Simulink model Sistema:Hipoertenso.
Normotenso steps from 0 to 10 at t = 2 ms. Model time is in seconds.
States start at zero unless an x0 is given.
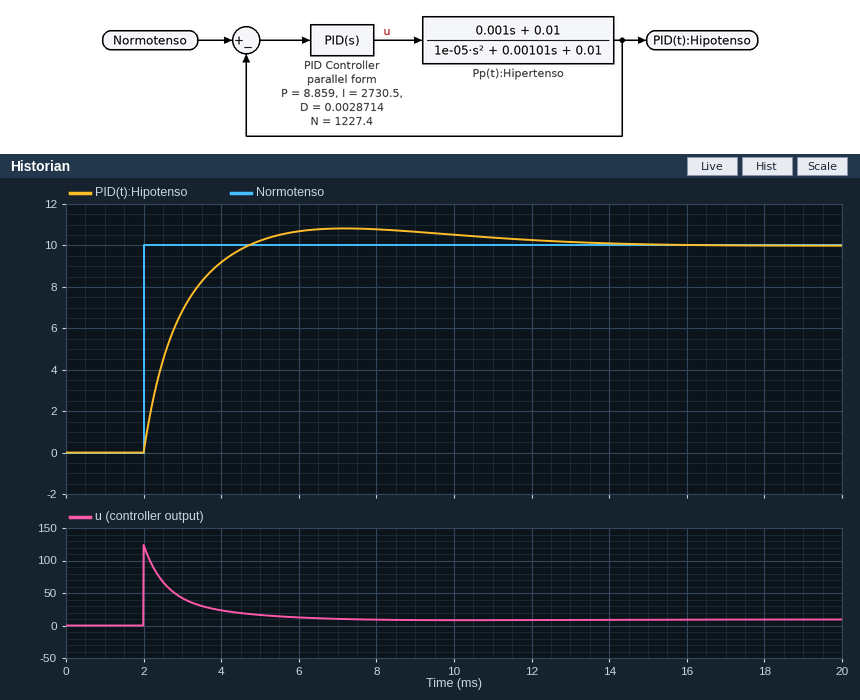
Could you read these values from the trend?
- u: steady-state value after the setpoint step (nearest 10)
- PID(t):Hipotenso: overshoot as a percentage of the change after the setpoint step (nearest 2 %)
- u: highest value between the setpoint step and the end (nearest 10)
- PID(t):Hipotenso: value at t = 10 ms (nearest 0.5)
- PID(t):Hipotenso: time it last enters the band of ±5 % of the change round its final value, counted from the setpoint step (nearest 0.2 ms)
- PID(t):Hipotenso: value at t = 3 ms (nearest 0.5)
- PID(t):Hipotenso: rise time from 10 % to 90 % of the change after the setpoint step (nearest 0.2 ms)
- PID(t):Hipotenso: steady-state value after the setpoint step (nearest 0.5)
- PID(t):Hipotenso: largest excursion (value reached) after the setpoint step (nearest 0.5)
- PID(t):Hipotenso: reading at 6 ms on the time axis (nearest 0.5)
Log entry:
10
8 %
120
10.5
8.2 ms
7.0
1.8 ms
10.0
11.0
10.5
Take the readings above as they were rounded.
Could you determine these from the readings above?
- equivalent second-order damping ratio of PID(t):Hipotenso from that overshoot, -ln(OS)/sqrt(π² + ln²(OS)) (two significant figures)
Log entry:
0.63
